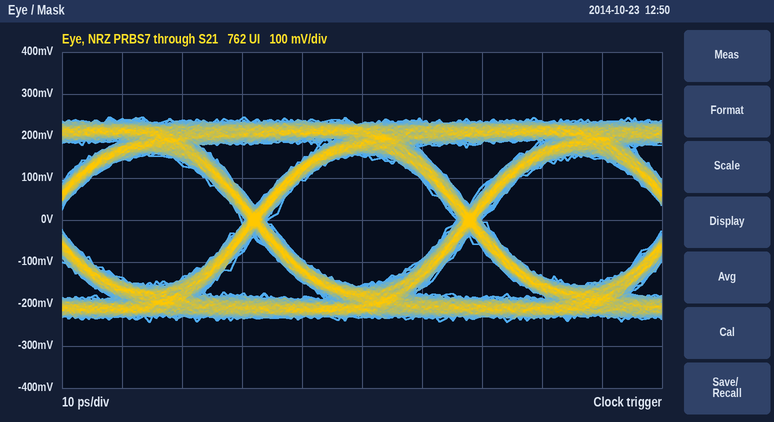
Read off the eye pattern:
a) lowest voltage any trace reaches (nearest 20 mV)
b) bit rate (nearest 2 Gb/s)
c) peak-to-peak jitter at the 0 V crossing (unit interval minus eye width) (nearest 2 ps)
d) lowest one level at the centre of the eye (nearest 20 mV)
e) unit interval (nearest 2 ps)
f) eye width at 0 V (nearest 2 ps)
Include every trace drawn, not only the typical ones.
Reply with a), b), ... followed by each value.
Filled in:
a) -240 mV
b) 28 Gb/s
c) 4 ps
d) 160 mV
e) 36 ps
f) 32 ps
